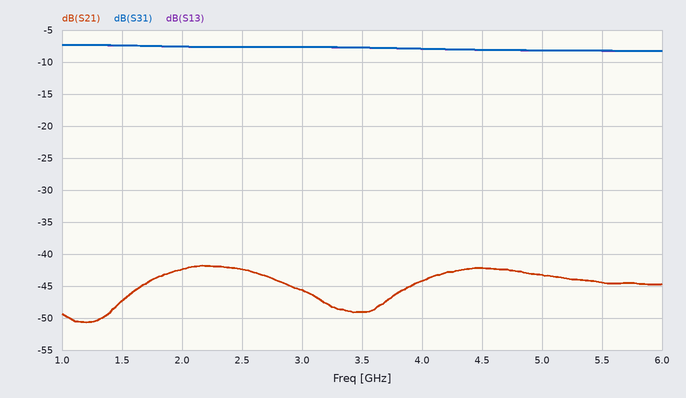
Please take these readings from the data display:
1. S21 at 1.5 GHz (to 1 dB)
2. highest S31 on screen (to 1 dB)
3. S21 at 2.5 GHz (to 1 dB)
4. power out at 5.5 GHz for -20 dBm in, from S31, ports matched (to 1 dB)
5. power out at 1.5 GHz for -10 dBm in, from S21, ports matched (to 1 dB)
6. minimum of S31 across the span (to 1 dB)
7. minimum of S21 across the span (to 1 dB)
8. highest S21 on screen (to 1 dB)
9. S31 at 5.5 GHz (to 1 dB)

-47 dB
-7 dB
-42 dB
-28 dBm
-57 dBm
-8 dB
-51 dB
-42 dB
-8 dB
